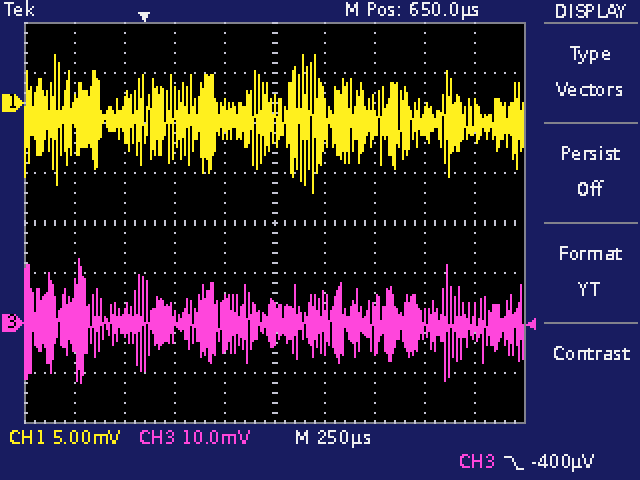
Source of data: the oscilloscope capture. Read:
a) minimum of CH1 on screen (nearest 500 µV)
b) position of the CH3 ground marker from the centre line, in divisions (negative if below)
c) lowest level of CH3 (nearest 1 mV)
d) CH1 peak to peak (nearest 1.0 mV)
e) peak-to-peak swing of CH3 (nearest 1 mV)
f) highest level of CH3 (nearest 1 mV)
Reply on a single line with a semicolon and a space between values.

-9.0 mV; -2.0 div; -12 mV; 14.0 mV; 25 mV; 13 mV
